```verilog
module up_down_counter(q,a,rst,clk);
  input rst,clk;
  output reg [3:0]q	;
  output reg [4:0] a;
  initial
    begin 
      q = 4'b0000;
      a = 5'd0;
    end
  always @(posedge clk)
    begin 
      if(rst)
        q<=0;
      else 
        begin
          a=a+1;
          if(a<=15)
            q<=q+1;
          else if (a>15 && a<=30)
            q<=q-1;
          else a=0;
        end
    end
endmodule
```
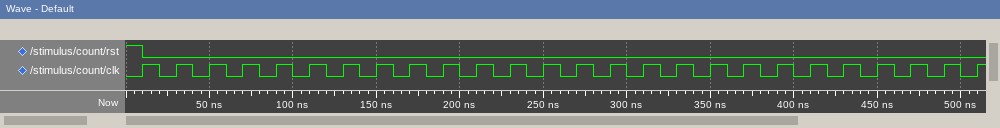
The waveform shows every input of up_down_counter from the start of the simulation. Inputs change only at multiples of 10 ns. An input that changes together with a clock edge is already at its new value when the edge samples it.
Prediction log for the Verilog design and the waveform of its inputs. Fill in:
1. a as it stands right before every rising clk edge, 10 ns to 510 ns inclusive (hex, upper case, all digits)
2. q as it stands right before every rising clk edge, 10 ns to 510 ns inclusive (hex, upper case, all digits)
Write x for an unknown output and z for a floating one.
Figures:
00, 01, 02, 03, 04, 05, 06, 07, 08, 09, 0A, 0B, 0C, 0D, 0E, 0F, 10, 11, 12, 13, 14, 15, 16, 17, 18, 19
0, 1, 2, 3, 4, 5, 6, 7, 8, 9, A, B, C, D, E, F, E, D, C, B, A, 9, 8, 7, 6, 5
